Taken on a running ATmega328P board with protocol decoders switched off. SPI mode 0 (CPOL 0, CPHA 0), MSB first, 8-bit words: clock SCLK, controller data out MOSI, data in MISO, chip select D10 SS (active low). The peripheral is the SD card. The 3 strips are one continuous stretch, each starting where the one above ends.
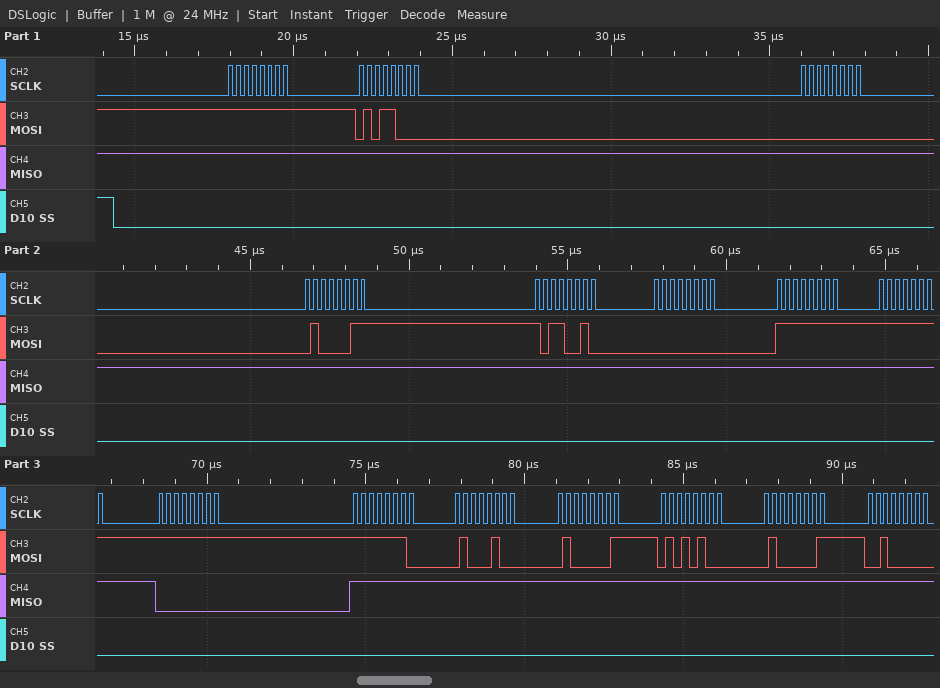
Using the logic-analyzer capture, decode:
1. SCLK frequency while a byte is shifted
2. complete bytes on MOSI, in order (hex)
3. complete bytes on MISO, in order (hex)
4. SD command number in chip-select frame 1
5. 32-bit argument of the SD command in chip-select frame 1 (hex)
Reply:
4 MHz
FF 58 00 43 B2 00 FF FF FF FE 44 41 54 41 20
FF FF FF FF FF FF FF FF 00 FF FF FF FF FF FF
CMD24
0x0043B200
